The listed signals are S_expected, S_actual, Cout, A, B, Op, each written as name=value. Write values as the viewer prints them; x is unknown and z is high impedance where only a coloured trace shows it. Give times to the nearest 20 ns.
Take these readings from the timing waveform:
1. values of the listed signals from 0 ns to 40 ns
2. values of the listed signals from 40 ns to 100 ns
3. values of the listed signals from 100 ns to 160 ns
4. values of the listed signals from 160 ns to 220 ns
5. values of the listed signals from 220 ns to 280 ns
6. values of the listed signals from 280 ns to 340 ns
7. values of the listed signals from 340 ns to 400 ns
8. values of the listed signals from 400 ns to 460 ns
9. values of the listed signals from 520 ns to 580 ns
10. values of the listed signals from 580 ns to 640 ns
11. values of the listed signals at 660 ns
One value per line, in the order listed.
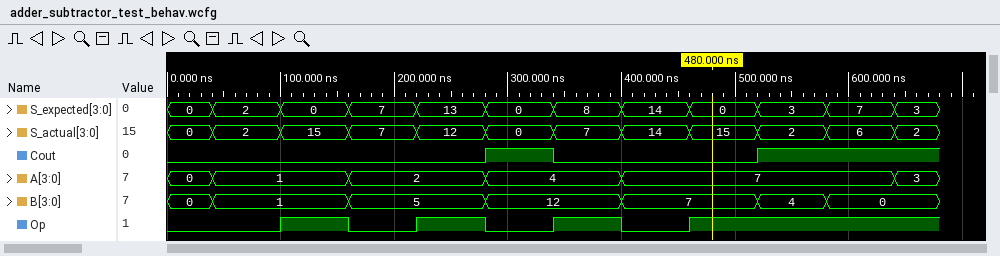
S_expected=0, S_actual=0, Cout=0, A=0, B=0, Op=0
S_expected=2, S_actual=2, Cout=0, A=1, B=1, Op=0
S_expected=0, S_actual=15, Cout=0, A=1, B=1, Op=1
S_expected=7, S_actual=7, Cout=0, A=2, B=5, Op=0
S_expected=13, S_actual=12, Cout=0, A=2, B=5, Op=1
S_expected=0, S_actual=0, Cout=1, A=4, B=12, Op=0
S_expected=8, S_actual=7, Cout=0, A=4, B=12, Op=1
S_expected=14, S_actual=14, Cout=0, A=7, B=7, Op=0
S_expected=3, S_actual=2, Cout=1, A=7, B=4, Op=1
S_expected=7, S_actual=6, Cout=1, A=7, B=0, Op=1
S_expected=3, S_actual=2, Cout=1, A=3, B=0, Op=1
